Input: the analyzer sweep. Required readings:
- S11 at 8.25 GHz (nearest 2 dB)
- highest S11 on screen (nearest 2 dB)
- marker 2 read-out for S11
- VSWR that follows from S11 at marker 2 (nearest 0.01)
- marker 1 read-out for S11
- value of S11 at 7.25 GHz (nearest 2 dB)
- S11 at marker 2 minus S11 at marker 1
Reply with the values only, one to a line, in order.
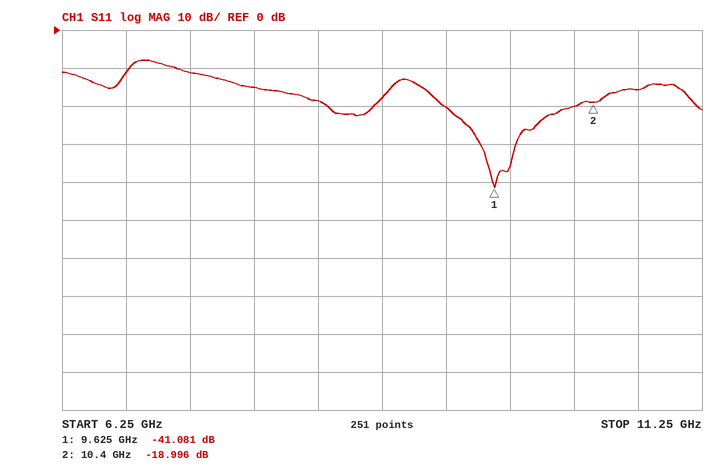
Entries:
-18 dB
-8 dB
-18.996 dB
1.25
-41.081 dB
-12 dB
22.085 dB
